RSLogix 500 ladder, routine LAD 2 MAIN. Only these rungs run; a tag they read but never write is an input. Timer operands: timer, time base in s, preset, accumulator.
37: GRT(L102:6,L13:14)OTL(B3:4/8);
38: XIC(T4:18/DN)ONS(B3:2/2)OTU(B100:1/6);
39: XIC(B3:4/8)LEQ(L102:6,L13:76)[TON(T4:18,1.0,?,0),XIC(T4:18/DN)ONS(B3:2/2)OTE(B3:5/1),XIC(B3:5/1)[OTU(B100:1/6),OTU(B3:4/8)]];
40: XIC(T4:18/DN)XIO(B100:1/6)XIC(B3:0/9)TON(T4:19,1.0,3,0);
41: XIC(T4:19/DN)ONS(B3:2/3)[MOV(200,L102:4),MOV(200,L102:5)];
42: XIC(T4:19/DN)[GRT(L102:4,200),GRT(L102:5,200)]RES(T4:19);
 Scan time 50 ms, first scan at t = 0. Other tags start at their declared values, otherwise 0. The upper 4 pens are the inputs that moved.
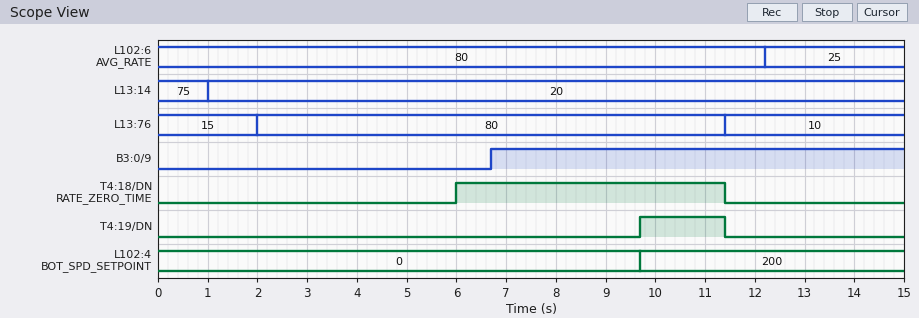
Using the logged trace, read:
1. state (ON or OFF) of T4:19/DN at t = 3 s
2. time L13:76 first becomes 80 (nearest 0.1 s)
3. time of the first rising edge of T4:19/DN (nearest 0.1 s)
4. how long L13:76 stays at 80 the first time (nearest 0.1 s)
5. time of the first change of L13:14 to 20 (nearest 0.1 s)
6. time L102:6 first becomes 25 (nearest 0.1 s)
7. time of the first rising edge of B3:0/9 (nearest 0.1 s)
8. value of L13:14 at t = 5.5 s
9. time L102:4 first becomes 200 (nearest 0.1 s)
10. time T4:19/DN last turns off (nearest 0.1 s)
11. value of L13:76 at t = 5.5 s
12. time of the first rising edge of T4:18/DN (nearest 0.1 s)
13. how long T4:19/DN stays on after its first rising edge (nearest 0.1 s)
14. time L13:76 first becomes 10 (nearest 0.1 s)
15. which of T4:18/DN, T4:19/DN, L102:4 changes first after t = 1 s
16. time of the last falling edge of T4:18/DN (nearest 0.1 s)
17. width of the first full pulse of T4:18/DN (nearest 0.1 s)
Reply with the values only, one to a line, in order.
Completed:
OFF
2.0 s
9.7 s
9.4 s
1.0 s
12.2 s
6.7 s
20
9.7 s
11.4 s
80
6.0 s
1.7 s
11.4 s
T4:18/DN
11.4 s
5.4 s
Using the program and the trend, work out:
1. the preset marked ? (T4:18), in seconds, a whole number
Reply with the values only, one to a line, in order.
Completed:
4 s
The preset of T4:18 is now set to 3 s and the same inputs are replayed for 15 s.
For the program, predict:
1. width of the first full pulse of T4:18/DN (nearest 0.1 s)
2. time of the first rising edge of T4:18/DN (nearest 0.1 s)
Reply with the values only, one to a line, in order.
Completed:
6.4 s
5.0 s
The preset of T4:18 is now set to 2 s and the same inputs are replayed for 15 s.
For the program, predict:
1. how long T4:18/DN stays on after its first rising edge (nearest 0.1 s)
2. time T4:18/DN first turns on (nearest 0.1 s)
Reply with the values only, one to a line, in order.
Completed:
7.4 s
4.0 s
